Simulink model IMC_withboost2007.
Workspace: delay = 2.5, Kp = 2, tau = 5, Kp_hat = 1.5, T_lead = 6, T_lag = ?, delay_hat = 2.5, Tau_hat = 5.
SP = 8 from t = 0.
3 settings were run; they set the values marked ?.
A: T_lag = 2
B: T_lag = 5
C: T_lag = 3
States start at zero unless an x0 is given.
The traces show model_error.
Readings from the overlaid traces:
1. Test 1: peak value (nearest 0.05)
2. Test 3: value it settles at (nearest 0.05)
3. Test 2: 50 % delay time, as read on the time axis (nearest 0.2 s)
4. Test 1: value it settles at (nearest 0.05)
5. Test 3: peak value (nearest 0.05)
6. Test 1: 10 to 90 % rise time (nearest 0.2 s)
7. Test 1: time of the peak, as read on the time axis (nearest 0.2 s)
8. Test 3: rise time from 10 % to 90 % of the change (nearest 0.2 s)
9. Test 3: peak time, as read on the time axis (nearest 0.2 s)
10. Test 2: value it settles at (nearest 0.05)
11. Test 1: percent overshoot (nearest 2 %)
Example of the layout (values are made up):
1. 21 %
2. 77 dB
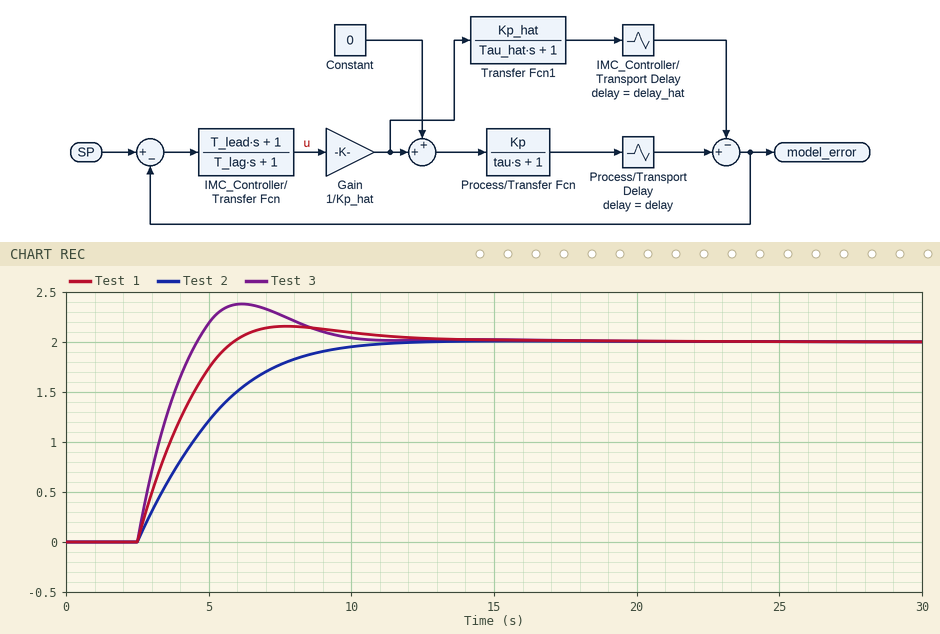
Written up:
1. 2.15
2. 2.00
3. 4.4 s
4. 2.00
5. 2.40
6. 2.4 s
7. 7.8 s
8. 1.6 s
9. 6.2 s
10. 2.00
11. 8 %
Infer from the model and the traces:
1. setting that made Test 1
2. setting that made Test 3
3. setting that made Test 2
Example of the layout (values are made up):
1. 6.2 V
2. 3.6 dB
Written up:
1. C
2. A
3. B
